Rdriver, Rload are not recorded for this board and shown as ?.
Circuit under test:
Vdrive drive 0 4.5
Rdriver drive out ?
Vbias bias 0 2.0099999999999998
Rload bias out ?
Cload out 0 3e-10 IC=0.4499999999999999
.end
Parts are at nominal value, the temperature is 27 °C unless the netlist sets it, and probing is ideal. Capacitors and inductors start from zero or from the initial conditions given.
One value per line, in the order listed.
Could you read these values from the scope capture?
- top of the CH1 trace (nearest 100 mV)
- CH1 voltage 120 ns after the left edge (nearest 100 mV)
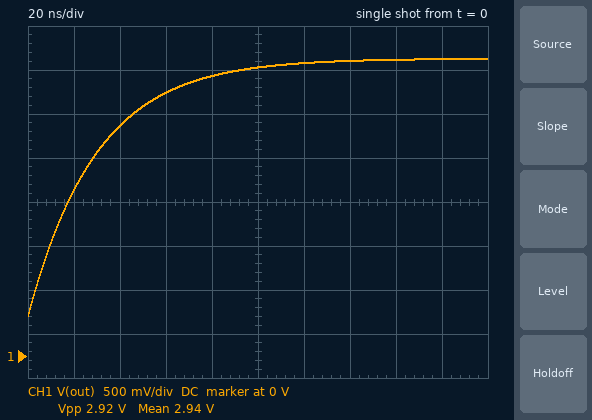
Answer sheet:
3.4 V
3.3 V
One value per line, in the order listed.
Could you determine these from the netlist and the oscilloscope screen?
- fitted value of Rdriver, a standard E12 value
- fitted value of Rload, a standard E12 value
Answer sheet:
180 Ω
220 Ω
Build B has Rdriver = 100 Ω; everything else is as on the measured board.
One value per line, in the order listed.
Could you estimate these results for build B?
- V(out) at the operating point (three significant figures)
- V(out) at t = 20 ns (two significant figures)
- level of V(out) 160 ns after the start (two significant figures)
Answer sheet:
3.72 V
2.5 V
3.7 V
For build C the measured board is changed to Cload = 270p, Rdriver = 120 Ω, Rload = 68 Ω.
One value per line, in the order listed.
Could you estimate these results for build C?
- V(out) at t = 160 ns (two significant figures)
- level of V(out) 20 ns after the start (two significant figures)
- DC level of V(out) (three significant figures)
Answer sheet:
2.9 V
2.5 V
2.91 V
